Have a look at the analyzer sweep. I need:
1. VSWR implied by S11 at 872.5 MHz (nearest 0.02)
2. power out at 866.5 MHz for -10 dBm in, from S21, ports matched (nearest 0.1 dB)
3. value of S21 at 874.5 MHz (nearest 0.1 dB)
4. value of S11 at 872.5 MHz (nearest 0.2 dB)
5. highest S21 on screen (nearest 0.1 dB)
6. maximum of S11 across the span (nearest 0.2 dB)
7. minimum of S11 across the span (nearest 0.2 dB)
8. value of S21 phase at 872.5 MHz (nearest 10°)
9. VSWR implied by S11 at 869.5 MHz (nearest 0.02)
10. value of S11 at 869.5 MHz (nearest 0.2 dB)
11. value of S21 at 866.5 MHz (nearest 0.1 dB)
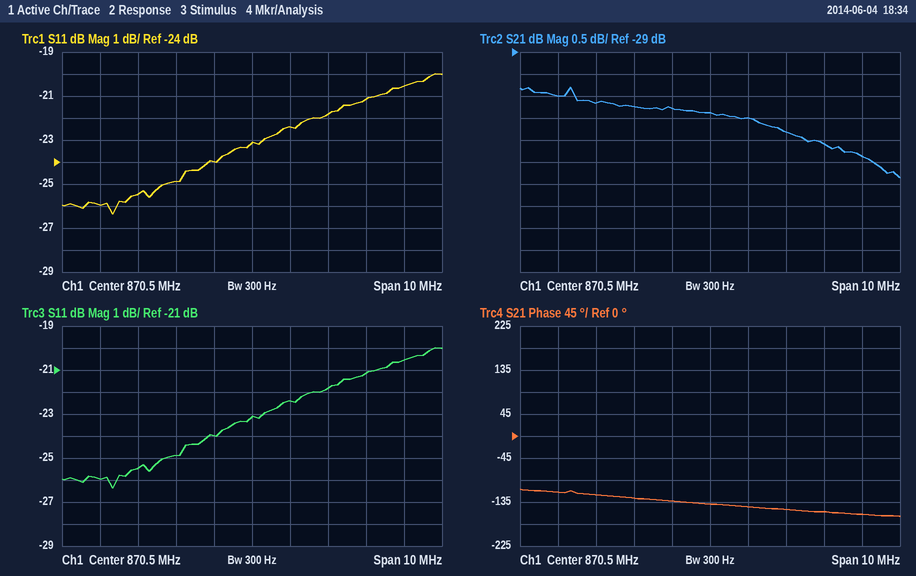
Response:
1.18
-40.0 dBm
-31.4 dB
-21.8 dB
-29.8 dB
-20.0 dB
-26.4 dB
-150°
1.14
-24.0 dB
-30.0 dB
